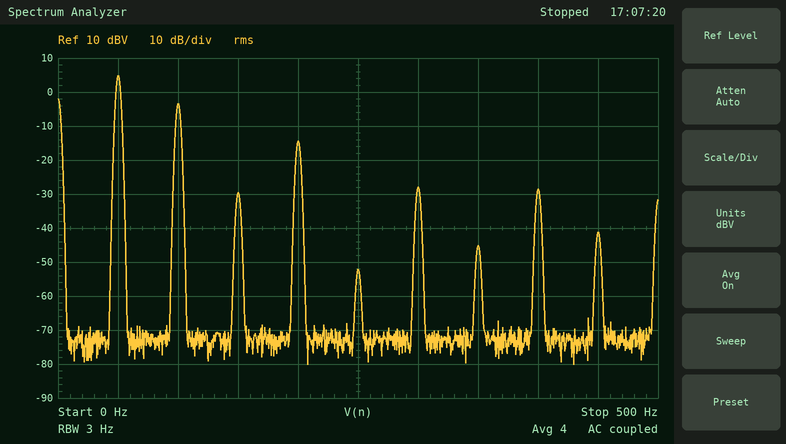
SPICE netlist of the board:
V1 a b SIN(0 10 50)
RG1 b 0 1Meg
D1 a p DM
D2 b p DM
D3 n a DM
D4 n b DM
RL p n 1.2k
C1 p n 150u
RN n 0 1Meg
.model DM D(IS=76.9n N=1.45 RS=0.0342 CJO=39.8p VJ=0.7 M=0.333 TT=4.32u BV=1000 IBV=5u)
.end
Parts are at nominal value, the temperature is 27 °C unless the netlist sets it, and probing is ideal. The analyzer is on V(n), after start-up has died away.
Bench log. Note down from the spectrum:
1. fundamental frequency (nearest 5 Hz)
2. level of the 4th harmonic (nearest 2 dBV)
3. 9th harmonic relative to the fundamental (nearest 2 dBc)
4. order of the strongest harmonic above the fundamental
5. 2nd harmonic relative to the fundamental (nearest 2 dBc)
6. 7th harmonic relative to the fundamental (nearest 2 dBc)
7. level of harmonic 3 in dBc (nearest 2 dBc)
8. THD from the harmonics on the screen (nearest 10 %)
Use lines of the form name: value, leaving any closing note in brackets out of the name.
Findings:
fundamental frequency: 50 Hz
level of the 4th harmonic: -14 dBV
9th harmonic relative to the fundamental: -46 dBc
order of the strongest harmonic above the fundamental: 2
2nd harmonic relative to the fundamental: -8 dBc
7th harmonic relative to the fundamental: -50 dBc
level of harmonic 3 in dBc: -34 dBc
THD from the harmonics on the screen: 40 %
